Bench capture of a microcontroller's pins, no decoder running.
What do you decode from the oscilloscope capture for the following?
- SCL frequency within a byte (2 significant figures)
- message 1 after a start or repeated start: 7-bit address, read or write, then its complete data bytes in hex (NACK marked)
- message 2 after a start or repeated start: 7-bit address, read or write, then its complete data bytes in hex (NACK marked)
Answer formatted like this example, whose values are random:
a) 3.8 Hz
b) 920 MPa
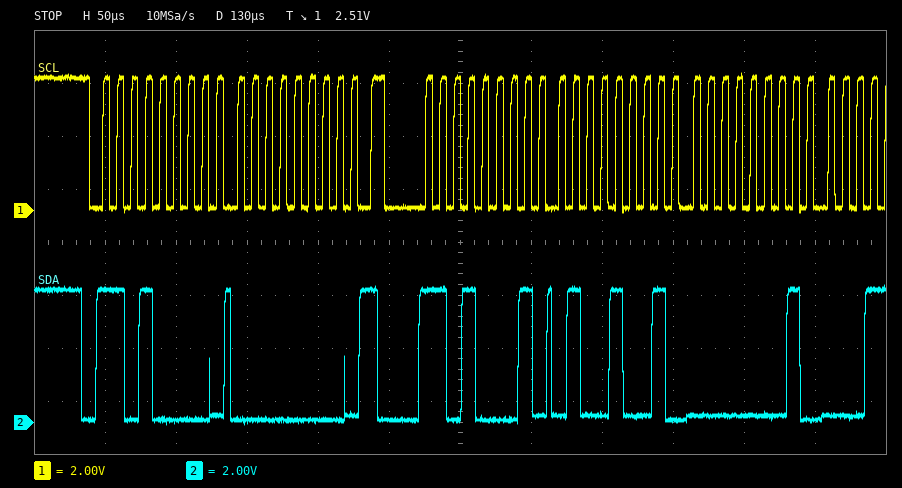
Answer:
a) 100 kHz
b) 0x68 write: 00
c) 0x68 read: 49 01
